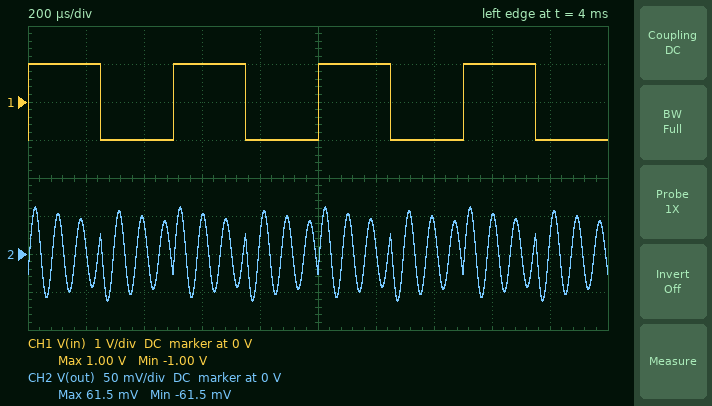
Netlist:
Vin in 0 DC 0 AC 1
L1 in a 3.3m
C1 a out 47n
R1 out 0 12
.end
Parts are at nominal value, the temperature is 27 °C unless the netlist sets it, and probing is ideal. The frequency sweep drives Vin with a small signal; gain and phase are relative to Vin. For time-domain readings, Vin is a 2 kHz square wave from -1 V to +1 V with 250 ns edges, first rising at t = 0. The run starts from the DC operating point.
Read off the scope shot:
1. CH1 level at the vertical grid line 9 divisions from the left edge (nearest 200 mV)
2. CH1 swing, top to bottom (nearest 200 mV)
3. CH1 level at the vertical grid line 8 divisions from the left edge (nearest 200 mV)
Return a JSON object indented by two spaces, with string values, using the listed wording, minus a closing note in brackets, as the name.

{
  "CH1 level at the vertical grid line 9 divisions from the left edge": "-1.0 V",
  "CH1 swing, top to bottom": "2.0 V",
  "CH1 level at the vertical grid line 8 divisions from the left edge": "1.0 V"
}
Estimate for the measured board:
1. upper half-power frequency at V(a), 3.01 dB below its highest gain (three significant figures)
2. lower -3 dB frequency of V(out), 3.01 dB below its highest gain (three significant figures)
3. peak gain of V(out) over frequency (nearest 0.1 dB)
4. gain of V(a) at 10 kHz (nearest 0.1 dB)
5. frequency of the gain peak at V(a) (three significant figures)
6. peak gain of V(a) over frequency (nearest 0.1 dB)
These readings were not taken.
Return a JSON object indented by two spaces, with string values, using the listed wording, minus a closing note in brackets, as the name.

{
  "upper half-power frequency at V(a), 3.01 dB below its highest gain": "13.1 kHz",
  "lower -3 dB frequency of V(out), 3.01 dB below its highest gain": "12.5 kHz",
  "peak gain of V(out) over frequency": "0 dB",
  "gain of V(a) at 10 kHz": "8.2 dB",
  "frequency of the gain peak at V(a)": "12.8 kHz",
  "peak gain of V(a) over frequency": "26.9 dB"
}
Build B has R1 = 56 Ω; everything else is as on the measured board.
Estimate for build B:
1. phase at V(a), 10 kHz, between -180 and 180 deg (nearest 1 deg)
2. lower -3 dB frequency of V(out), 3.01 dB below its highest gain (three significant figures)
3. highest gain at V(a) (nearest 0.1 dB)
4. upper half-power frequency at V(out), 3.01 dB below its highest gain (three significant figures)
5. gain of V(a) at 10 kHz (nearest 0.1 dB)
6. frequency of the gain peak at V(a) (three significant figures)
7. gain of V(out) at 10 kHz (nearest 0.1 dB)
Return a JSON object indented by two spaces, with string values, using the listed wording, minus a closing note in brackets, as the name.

{
  "phase at V(a), 10 kHz, between -180 and 180 deg": "-14 deg",
  "lower -3 dB frequency of V(out), 3.01 dB below its highest gain": "11.5 kHz",
  "highest gain at V(a)": "13.7 dB",
  "upper half-power frequency at V(out), 3.01 dB below its highest gain": "14.2 kHz",
  "gain of V(a) at 10 kHz": "7.6 dB",
  "frequency of the gain peak at V(a)": "12.6 kHz",
  "gain of V(out) at 10 kHz": "-8.1 dB"
}
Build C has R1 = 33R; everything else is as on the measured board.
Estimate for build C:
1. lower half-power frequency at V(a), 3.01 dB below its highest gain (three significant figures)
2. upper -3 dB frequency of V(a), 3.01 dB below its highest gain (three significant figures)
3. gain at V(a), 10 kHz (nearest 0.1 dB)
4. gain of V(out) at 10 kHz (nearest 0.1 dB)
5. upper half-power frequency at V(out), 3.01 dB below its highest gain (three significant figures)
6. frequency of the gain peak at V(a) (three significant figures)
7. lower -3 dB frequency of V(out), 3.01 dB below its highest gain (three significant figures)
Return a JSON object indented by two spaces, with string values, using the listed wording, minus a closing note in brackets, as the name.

{
  "lower half-power frequency at V(a), 3.01 dB below its highest gain": "11.9 kHz",
  "upper -3 dB frequency of V(a), 3.01 dB below its highest gain": "13.5 kHz",
  "gain at V(a), 10 kHz": "8.0 dB",
  "gain of V(out) at 10 kHz": "-12.3 dB",
  "upper half-power frequency at V(out), 3.01 dB below its highest gain": "13.6 kHz",
  "frequency of the gain peak at V(a)": "12.7 kHz",
  "lower -3 dB frequency of V(out), 3.01 dB below its highest gain": "12.0 kHz"
}
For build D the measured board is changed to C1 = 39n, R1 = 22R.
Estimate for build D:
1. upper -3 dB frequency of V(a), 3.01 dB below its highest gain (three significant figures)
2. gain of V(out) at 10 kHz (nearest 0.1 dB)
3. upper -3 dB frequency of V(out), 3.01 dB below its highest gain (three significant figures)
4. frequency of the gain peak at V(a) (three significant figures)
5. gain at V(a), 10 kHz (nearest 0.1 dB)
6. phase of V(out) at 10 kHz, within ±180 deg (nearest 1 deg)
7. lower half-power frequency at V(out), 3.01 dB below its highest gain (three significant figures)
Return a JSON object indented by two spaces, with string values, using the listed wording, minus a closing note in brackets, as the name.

{
  "upper -3 dB frequency of V(a), 3.01 dB below its highest gain": "14.5 kHz",
  "gain of V(out) at 10 kHz": "-19.3 dB",
  "upper -3 dB frequency of V(out), 3.01 dB below its highest gain": "14.6 kHz",
  "frequency of the gain peak at V(a)": "14.0 kHz",
  "gain at V(a), 10 kHz": "6.1 dB",
  "phase of V(out) at 10 kHz, within ±180 deg": "84 deg",
  "lower half-power frequency at V(out), 3.01 dB below its highest gain": "13.5 kHz"
}
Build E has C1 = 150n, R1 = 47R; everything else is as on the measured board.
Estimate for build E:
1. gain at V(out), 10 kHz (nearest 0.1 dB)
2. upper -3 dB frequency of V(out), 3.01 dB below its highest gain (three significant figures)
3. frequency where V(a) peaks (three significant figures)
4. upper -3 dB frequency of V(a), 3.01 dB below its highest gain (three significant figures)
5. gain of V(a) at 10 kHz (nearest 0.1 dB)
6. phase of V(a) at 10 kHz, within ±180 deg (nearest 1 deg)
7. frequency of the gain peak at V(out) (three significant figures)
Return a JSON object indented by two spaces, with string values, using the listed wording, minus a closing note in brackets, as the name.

{
  "gain at V(out), 10 kHz": "-7.5 dB",
  "upper -3 dB frequency of V(out), 3.01 dB below its highest gain": "8.38 kHz",
  "frequency where V(a) peaks": "6.99 kHz",
  "upper -3 dB frequency of V(a), 3.01 dB below its highest gain": "8.07 kHz",
  "gain of V(a) at 10 kHz": "0.3 dB",
  "phase of V(a) at 10 kHz, within ±180 deg": "-131 deg",
  "frequency of the gain peak at V(out)": "7.15 kHz"
}
